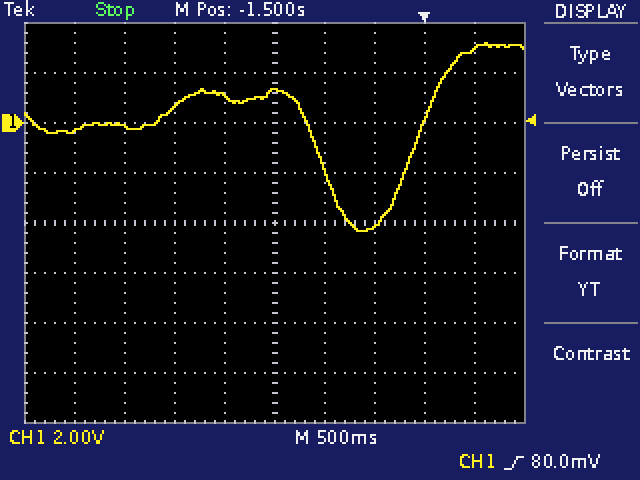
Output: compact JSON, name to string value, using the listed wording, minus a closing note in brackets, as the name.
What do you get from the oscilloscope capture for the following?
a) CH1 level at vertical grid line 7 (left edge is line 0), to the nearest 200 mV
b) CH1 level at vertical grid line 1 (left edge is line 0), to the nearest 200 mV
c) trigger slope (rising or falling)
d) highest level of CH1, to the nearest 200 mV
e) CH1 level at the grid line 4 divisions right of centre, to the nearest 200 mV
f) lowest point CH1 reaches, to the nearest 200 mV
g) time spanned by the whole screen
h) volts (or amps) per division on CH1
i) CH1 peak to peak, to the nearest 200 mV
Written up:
{"CH1 level at vertical grid line 7 (left edge is line 0), to the nearest 200 mV": "-4.2 V", "CH1 level at vertical grid line 1 (left edge is line 0), to the nearest 200 mV": "-400 mV", "trigger slope": "rising", "highest level of CH1, to the nearest 200 mV": "3.2 V", "CH1 level at the grid line 4 divisions right of centre, to the nearest 200 mV": "3.0 V", "lowest point CH1 reaches, to the nearest 200 mV": "-4.4 V", "time spanned by the whole screen": "5 s", "volts (or amps) per division on CH1": "2 V", "CH1 peak to peak, to the nearest 200 mV": "7.6 V"}
